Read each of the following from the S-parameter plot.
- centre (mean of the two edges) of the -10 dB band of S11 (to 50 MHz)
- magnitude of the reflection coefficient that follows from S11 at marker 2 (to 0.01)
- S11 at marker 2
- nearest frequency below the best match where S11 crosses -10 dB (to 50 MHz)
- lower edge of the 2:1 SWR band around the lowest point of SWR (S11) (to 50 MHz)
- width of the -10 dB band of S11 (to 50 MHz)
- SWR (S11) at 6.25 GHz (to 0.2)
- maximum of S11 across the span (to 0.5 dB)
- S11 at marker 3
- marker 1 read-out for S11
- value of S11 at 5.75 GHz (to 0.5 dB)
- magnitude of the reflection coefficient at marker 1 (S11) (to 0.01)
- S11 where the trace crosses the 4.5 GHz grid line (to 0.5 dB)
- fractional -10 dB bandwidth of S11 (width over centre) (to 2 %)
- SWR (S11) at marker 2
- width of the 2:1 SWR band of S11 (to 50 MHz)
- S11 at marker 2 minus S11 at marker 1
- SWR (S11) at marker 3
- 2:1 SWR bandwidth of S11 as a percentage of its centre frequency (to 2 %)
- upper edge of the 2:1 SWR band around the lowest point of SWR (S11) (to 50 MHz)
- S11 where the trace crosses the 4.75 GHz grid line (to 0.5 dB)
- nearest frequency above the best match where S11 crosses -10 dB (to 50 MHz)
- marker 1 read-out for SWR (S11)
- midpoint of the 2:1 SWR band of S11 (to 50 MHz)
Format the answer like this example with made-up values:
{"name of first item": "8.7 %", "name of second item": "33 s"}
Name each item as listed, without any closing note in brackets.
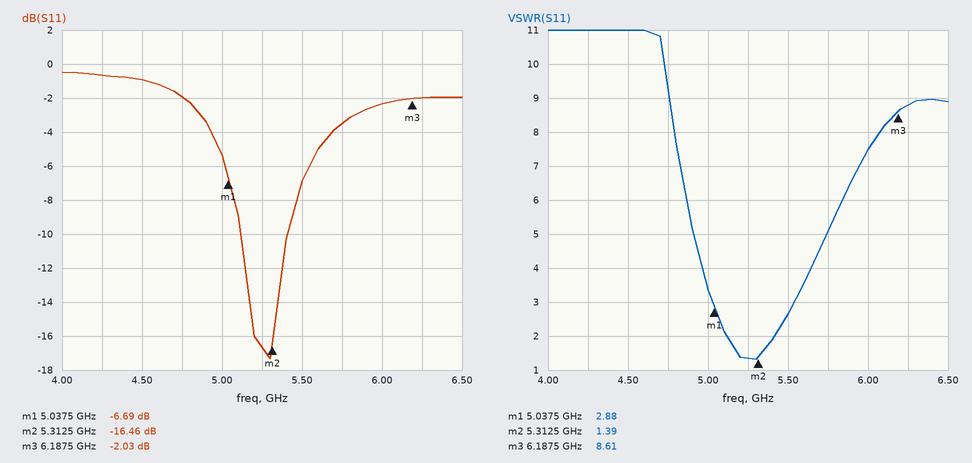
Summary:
{"centre (mean of the two edges) of the -10 dB band of S11": "5.25 GHz", "magnitude of the reflection coefficient that follows from S11 at marker 2": "0.15", "S11 at marker 2": "-16.46 dB", "nearest frequency below the best match where S11 crosses -10 dB": "5.10 GHz", "lower edge of the 2:1 SWR band around the lowest point of SWR (S11)": "5.10 GHz", "width of the -10 dB band of S11": "300 MHz", "SWR (S11) at 6.25 GHz": "8.8", "maximum of S11 across the span": "-0.5 dB", "S11 at marker 3": "-2.03 dB", "marker 1 read-out for S11": "-6.69 dB", "value of S11 at 5.75 GHz": "-3.5 dB", "magnitude of the reflection coefficient at marker 1 (S11)": "0.46", "S11 where the trace crosses the 4.5 GHz grid line": "-1.0 dB", "fractional -10 dB bandwidth of S11 (width over centre)": "6 %", "SWR (S11) at marker 2": "1.39", "width of the 2:1 SWR band of S11": "300 MHz", "S11 at marker 2 minus S11 at marker 1": "-9.77 dB", "SWR (S11) at marker 3": "8.61", "2:1 SWR bandwidth of S11 as a percentage of its centre frequency": "6 %", "upper edge of the 2:1 SWR band around the lowest point of SWR (S11)": "5.40 GHz", "S11 where the trace crosses the 4.75 GHz grid line": "-2.0 dB", "nearest frequency above the best match where S11 crosses -10 dB": "5.40 GHz", "marker 1 read-out for SWR": "2.88", "midpoint of the 2:1 SWR band of S11": "5.25 GHz"}
